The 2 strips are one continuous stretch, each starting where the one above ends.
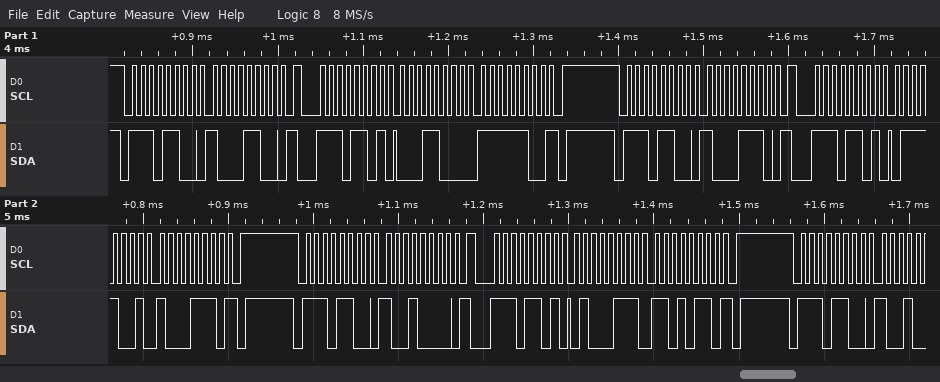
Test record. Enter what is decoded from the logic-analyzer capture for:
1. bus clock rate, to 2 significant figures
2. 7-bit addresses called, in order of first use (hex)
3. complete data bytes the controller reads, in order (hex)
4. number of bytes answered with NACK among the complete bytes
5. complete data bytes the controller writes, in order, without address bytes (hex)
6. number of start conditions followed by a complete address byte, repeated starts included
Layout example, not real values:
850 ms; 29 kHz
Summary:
100 kHz; 0x76; 18 FC 79 8E 47 D6; 3; 8C 8E 90; 7
